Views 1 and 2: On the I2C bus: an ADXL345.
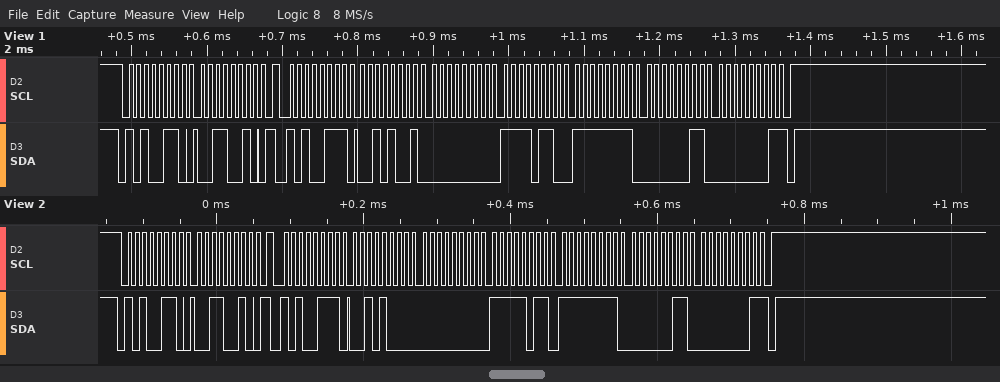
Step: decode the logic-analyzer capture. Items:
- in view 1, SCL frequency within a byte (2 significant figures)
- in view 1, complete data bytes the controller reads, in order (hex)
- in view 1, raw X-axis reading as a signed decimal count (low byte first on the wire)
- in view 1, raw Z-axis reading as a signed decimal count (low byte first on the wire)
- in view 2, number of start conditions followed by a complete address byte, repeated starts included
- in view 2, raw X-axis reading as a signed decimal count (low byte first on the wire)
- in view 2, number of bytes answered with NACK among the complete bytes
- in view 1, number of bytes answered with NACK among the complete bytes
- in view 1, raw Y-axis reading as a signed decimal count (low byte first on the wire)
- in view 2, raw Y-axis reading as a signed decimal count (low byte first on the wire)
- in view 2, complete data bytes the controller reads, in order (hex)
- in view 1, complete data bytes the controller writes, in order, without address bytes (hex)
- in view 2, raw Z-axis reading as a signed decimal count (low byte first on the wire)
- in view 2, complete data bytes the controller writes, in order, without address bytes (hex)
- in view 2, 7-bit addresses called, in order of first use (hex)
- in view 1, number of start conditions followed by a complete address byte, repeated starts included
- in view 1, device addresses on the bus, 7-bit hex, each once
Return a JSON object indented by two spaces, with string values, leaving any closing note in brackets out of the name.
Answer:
{
  "in view 1, SCL frequency within a byte": "100 kHz",
  "in view 1, complete data bytes the controller reads, in order": "29 00 F6 FF 03 01",
  "in view 1, raw X-axis reading as a signed decimal count": "41",
  "in view 1, raw Z-axis reading as a signed decimal count": "259",
  "in view 2, number of start conditions followed by a complete address byte, repeated starts included": "2",
  "in view 2, raw X-axis reading as a signed decimal count": "40",
  "in view 2, number of bytes answered with NACK among the complete bytes": "1",
  "in view 1, number of bytes answered with NACK among the complete bytes": "1",
  "in view 1, raw Y-axis reading as a signed decimal count": "-10",
  "in view 2, raw Y-axis reading as a signed decimal count": "-5",
  "in view 2, complete data bytes the controller reads, in order": "28 00 FB FF 03 01",
  "in view 1, complete data bytes the controller writes, in order, without address bytes": "32",
  "in view 2, raw Z-axis reading as a signed decimal count": "259",
  "in view 2, complete data bytes the controller writes, in order, without address bytes": "32",
  "in view 2, 7-bit addresses called, in order of first use": "0x53",
  "in view 1, number of start conditions followed by a complete address byte, repeated starts included": "2",
  "in view 1, device addresses on the bus, 7-bit hex, each once": "0x53"
}
